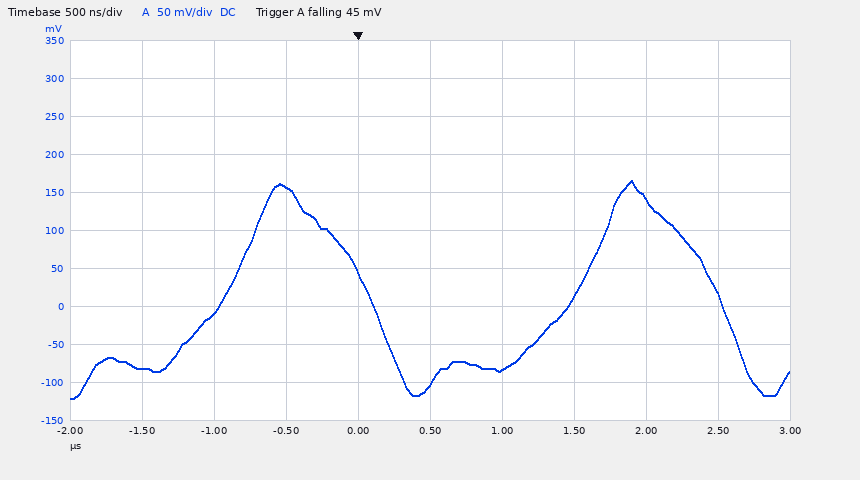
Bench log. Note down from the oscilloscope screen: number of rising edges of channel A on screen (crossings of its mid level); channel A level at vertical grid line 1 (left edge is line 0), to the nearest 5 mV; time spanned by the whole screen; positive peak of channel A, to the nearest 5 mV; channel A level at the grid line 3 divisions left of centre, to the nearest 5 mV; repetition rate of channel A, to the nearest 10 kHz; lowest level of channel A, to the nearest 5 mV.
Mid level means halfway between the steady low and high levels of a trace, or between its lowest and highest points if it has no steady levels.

2
-80 mV
5 µs
165 mV
-10 mV
410 kHz
-120 mV
